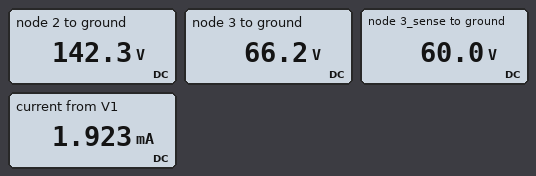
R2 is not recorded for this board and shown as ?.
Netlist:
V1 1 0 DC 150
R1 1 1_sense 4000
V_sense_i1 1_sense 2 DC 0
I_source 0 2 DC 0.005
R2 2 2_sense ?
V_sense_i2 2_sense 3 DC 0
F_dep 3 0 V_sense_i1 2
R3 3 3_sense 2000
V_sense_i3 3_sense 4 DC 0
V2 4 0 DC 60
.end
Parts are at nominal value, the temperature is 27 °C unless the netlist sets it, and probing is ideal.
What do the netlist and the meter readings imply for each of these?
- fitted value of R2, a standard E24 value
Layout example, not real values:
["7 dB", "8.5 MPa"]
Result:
["11 kΩ"]
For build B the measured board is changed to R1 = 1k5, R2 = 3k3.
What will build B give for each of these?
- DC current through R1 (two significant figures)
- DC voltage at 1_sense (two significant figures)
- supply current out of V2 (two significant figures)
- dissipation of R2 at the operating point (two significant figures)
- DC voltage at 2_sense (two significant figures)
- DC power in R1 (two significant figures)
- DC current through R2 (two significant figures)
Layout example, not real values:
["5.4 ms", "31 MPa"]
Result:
["23 mA", "120 V", "18 mA", "2.5 W", "25 V", "770 mW", "28 mA"]
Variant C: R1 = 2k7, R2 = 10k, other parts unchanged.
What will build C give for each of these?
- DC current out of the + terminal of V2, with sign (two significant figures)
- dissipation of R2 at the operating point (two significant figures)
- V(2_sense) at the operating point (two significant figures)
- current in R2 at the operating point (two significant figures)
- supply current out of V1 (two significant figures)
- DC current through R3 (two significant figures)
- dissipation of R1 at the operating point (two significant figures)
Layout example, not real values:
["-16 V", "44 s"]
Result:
["-2.2 mA", "610 mW", "64 V", "7.8 mA", "2.8 mA", "2.2 mA", "21 mW"]
